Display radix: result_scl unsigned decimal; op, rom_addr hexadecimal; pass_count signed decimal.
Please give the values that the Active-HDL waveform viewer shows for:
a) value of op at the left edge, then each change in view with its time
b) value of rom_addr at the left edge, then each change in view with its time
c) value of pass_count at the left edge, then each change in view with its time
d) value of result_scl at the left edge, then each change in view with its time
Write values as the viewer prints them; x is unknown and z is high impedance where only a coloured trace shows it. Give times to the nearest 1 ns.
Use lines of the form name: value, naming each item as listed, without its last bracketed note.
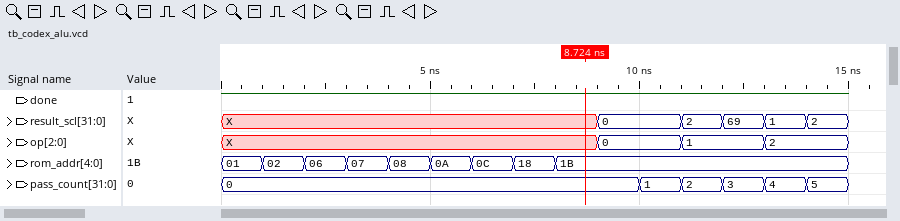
value of op at the left edge, then each change in view with its time: X, 0 at 9 ns, 1 at 11 ns, 2 at 13 ns
value of rom_addr at the left edge, then each change in view with its time: 01, 02 at 1 ns, 06 at 2 ns, 07 at 3 ns, 08 at 4 ns, 0A at 5 ns, 0C at 6 ns, 18 at 7 ns, 1B at 8 ns
value of pass_count at the left edge, then each change in view with its time: 0, 1 at 10 ns, 2 at 11 ns, 3 at 12 ns, 4 at 13 ns, 5 at 14 ns
value of result_scl at the left edge, then each change in view with its time: X, 0 at 9 ns, 2 at 11 ns, 69 at 12 ns, 1 at 13 ns, 2 at 14 ns
